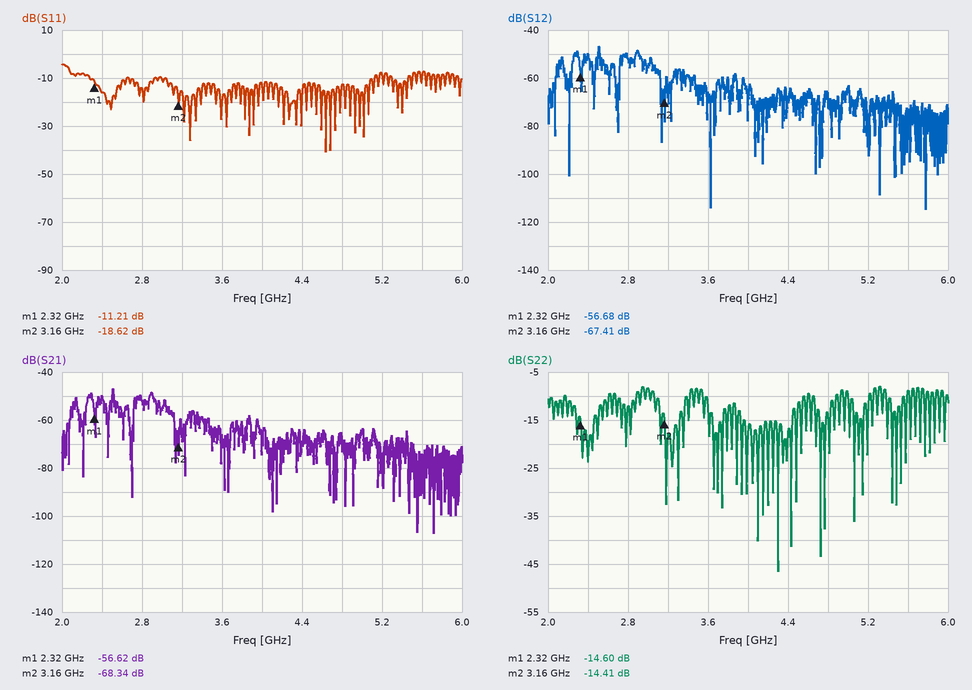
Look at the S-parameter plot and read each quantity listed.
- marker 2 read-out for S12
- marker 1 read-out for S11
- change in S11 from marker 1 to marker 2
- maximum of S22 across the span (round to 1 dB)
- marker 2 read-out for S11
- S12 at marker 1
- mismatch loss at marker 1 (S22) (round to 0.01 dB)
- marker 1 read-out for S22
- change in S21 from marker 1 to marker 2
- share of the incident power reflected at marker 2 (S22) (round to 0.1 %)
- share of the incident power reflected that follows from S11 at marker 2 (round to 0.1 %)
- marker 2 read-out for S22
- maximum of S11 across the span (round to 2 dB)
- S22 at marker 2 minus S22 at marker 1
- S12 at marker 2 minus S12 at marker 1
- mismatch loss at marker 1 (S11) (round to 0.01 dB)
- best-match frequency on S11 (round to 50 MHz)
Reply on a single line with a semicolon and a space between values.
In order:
-67.41 dB; -11.21 dB; -7.41 dB; -8 dB; -18.62 dB; -56.68 dB; 0.15 dB; -14.60 dB; -11.72 dB; 3.6 %; 1.4 %; -14.41 dB; -4 dB; 0.19 dB; -10.73 dB; 0.34 dB; 4.65 GHz
